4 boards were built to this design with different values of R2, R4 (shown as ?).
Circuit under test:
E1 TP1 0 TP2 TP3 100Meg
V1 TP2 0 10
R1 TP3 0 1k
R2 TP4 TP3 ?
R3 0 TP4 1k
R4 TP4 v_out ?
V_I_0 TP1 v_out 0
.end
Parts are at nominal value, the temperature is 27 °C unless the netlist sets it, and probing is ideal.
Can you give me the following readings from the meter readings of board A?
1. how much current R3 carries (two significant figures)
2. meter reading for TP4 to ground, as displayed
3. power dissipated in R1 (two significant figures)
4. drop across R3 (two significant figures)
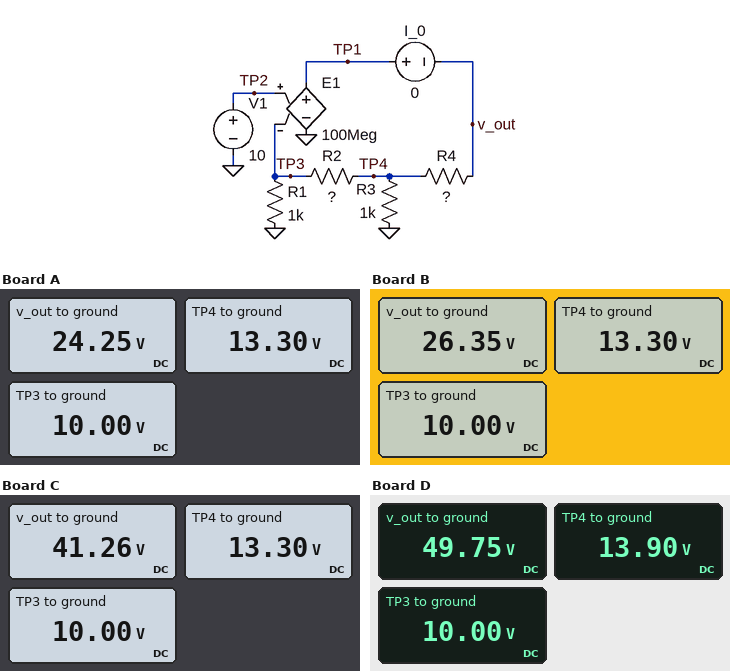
13 mA
13.30 V
100 mW
13 V
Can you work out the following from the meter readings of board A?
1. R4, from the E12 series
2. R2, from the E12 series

470 Ω
330 Ω
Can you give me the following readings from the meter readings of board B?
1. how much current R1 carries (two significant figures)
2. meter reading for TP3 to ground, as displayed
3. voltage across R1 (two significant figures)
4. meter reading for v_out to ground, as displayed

10 mA
10.00 V
10 V
26.35 V
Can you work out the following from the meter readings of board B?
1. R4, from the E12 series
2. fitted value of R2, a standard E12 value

560 Ω
330 Ω
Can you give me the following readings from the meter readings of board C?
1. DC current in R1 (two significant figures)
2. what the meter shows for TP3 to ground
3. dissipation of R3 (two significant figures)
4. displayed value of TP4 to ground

10 mA
10.00 V
180 mW
13.30 V
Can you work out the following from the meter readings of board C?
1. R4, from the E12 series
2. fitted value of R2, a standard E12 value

1.2 kΩ
330 Ω
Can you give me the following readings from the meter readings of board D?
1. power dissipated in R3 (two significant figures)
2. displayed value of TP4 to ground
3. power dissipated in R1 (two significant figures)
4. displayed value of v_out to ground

190 mW
13.90 V
100 mW
49.75 V
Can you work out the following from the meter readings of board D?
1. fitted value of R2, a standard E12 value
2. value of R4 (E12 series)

390 Ω
1.5 kΩ
